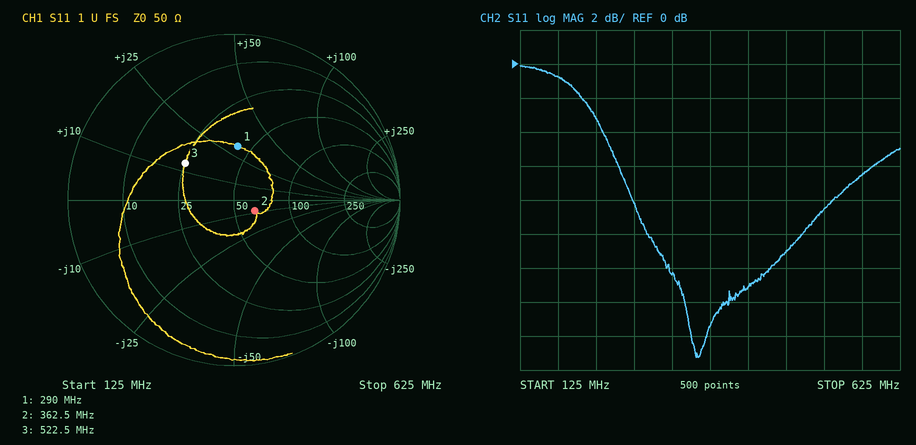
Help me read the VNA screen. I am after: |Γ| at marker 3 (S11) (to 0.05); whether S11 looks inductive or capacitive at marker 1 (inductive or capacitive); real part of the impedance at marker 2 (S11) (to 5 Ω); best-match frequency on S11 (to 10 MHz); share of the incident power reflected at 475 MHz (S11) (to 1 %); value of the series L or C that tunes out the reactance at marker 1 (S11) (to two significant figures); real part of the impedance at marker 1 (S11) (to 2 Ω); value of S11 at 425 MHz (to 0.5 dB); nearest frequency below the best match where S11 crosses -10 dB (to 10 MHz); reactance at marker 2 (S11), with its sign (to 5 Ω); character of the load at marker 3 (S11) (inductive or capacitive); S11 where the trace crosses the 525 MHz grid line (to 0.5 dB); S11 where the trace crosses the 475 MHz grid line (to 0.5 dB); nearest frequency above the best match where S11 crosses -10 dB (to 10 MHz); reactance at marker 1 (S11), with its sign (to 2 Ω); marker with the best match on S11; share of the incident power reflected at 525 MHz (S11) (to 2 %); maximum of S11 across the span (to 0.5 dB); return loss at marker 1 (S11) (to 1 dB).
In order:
0.35
inductive
65 Ω
360 MHz
8 %
18 pF
42 Ω
-13.0 dB
290 MHz
-10 Ω
inductive
-8.5 dB
-11.0 dB
500 MHz
+30 Ω
marker 2
14 %
0.0 dB
10 dB
